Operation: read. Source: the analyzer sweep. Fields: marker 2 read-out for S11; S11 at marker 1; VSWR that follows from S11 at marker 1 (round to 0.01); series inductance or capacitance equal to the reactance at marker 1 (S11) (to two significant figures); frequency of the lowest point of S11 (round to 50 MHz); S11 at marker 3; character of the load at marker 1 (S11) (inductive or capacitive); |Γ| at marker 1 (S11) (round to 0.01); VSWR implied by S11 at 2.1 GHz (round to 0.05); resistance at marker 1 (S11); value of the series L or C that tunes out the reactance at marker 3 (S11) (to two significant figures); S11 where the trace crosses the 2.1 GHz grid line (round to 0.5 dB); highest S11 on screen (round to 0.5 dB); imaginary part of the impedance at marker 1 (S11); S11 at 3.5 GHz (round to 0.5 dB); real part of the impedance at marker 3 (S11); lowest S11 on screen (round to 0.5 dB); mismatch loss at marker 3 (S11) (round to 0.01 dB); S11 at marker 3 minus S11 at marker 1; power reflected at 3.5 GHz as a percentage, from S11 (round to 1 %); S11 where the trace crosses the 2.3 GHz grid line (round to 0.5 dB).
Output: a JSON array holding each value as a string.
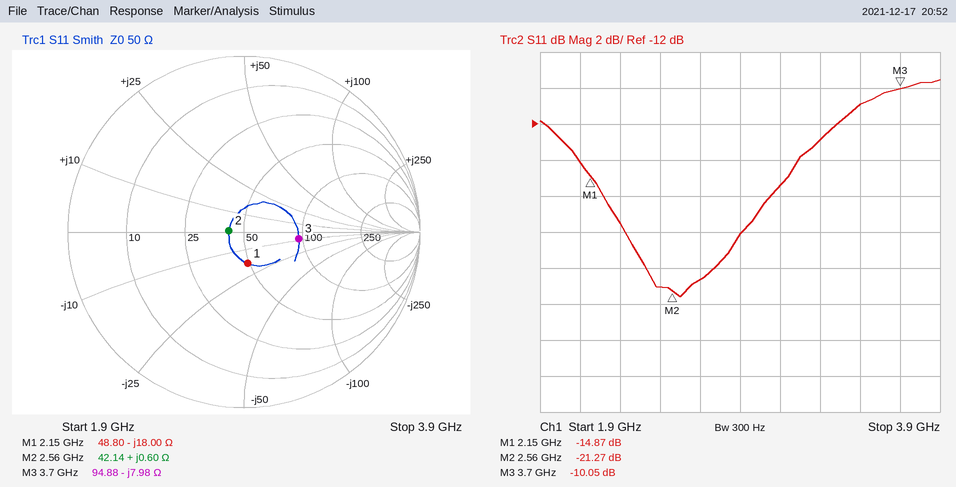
["-21.27 dB", "-14.87 dB", "1.44", "4.1 pF", "2.60 GHz", "-10.05 dB", "capacitive", "0.18", "1.50", "48.80 Ω", "340 pH", "-14.0 dB", "-9.5 dB", "-18.00 Ω", "-11.0 dB", "94.88 Ω", "-21.5 dB", "0.45 dB", "4.82 dB", "8 %", "-17.5 dB"]
